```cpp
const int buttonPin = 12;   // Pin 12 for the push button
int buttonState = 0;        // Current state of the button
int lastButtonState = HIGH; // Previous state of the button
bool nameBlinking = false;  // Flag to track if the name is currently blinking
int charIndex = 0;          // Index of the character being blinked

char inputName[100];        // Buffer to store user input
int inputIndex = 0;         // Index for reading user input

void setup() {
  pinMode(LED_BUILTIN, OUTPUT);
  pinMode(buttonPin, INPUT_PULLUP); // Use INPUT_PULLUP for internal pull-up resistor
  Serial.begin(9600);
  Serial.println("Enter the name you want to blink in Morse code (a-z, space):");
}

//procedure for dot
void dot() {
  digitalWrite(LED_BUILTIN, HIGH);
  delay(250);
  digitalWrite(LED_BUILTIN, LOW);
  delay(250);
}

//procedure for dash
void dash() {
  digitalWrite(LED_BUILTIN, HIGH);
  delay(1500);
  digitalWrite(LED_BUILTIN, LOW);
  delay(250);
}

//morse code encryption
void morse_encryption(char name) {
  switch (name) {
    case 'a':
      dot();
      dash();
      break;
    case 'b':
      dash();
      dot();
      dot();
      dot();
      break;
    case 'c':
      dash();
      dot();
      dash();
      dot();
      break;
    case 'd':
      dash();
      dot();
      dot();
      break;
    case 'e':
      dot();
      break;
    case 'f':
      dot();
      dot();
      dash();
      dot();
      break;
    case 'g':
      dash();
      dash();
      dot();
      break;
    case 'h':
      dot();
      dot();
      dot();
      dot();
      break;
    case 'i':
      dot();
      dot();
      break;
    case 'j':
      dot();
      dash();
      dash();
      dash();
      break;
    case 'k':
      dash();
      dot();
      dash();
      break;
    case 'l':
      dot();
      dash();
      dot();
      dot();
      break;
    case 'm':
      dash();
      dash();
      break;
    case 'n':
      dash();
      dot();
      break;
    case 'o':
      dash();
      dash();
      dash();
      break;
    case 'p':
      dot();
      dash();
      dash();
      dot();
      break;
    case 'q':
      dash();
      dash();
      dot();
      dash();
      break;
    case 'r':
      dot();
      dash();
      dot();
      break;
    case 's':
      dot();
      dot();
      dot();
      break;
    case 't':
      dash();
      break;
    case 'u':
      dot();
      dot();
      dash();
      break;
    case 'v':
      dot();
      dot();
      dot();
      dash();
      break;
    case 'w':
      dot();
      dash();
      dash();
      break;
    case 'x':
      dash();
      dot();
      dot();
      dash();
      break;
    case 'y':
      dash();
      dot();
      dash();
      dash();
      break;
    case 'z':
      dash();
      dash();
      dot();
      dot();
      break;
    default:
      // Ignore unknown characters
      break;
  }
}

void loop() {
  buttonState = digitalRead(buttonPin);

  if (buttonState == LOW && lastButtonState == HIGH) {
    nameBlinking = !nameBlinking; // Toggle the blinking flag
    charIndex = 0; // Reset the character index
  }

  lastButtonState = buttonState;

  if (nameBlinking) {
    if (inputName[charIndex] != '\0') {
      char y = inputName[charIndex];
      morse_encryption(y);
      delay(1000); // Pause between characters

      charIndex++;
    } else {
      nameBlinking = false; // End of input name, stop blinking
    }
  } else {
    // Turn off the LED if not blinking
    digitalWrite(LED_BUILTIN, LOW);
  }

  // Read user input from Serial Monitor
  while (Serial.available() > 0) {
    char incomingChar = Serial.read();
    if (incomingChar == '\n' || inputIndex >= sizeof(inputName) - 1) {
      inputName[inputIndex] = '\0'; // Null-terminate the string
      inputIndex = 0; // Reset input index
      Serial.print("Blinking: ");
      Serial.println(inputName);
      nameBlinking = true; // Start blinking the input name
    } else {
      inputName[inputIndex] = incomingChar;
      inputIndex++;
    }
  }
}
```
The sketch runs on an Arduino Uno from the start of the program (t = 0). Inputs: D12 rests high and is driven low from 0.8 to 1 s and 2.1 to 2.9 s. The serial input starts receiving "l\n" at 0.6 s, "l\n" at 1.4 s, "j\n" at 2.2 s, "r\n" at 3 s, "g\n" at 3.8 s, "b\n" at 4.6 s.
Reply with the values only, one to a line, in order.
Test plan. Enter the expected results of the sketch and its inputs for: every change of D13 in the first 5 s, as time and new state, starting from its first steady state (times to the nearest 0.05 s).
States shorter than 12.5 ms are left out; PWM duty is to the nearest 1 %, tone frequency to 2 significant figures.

0 s low; 0.6 s high; 0.85 s low; 1.1 s high; 2.6 s low; 2.85 s high; 3.1 s low; 3.35 s high; 3.6 s low
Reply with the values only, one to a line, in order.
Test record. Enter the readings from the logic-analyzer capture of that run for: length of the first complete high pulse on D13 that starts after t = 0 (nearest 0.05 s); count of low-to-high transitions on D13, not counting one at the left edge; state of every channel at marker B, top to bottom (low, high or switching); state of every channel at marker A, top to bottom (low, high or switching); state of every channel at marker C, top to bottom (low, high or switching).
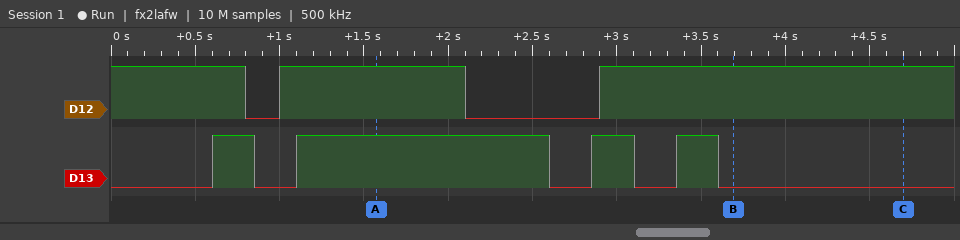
0.25 s
4
D12 high, D13 low
D12 high, D13 high
D12 high, D13 low
